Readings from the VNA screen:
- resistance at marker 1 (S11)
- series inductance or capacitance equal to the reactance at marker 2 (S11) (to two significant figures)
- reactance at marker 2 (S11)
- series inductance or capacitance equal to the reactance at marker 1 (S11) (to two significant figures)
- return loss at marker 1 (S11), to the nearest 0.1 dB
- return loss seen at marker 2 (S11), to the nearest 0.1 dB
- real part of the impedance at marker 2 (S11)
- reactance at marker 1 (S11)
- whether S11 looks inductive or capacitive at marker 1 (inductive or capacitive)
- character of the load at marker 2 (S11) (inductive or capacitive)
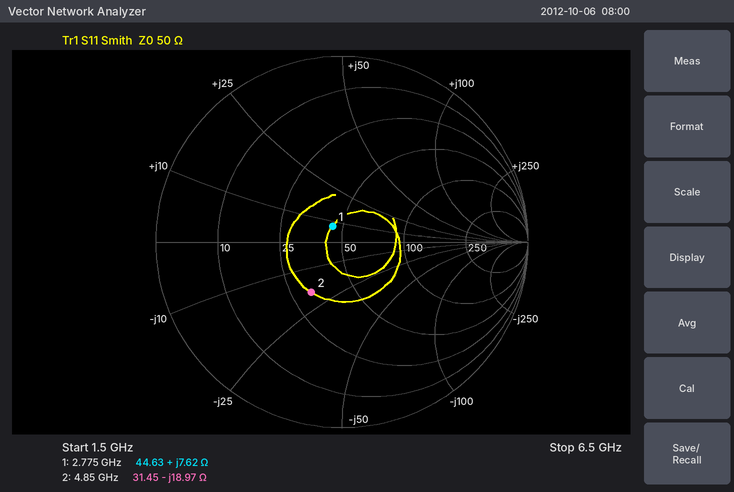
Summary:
44.63 Ω
1.7 pF
-18.97 Ω
440 pH
20.2 dB
10.0 dB
31.45 Ω
+7.62 Ω
inductive
capacitive
